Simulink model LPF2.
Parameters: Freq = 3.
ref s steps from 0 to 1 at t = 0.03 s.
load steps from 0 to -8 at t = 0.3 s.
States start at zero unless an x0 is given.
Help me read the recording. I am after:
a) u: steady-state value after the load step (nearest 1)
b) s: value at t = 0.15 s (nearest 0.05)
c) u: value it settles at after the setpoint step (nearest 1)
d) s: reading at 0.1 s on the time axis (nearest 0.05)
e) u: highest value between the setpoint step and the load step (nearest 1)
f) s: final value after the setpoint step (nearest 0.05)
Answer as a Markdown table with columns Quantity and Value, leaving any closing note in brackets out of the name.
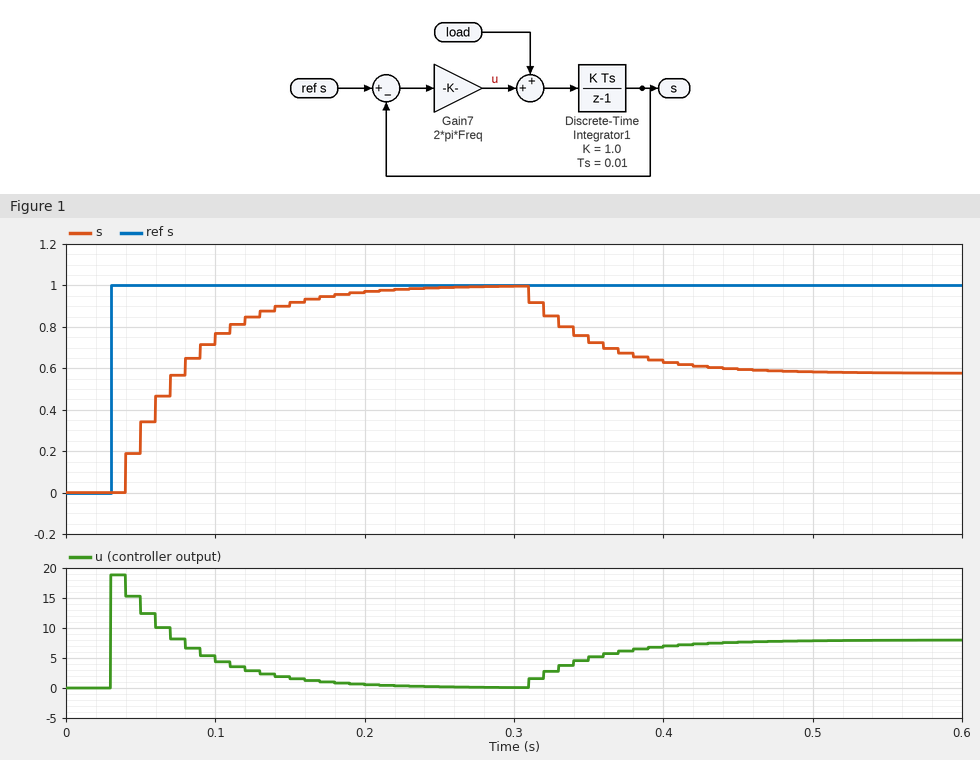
| Quantity | Value |
|---|---|
| u: steady-state value after the load step | 8 |
| s: value at t = 0.15 s | 0.90 |
| u: value it settles at after the setpoint step | 0 |
| s: reading at 0.1 s on the time axis | 0.75 |
| u: highest value between the setpoint step and the load step | 19 |
| s: final value after the setpoint step | 1.00 |
